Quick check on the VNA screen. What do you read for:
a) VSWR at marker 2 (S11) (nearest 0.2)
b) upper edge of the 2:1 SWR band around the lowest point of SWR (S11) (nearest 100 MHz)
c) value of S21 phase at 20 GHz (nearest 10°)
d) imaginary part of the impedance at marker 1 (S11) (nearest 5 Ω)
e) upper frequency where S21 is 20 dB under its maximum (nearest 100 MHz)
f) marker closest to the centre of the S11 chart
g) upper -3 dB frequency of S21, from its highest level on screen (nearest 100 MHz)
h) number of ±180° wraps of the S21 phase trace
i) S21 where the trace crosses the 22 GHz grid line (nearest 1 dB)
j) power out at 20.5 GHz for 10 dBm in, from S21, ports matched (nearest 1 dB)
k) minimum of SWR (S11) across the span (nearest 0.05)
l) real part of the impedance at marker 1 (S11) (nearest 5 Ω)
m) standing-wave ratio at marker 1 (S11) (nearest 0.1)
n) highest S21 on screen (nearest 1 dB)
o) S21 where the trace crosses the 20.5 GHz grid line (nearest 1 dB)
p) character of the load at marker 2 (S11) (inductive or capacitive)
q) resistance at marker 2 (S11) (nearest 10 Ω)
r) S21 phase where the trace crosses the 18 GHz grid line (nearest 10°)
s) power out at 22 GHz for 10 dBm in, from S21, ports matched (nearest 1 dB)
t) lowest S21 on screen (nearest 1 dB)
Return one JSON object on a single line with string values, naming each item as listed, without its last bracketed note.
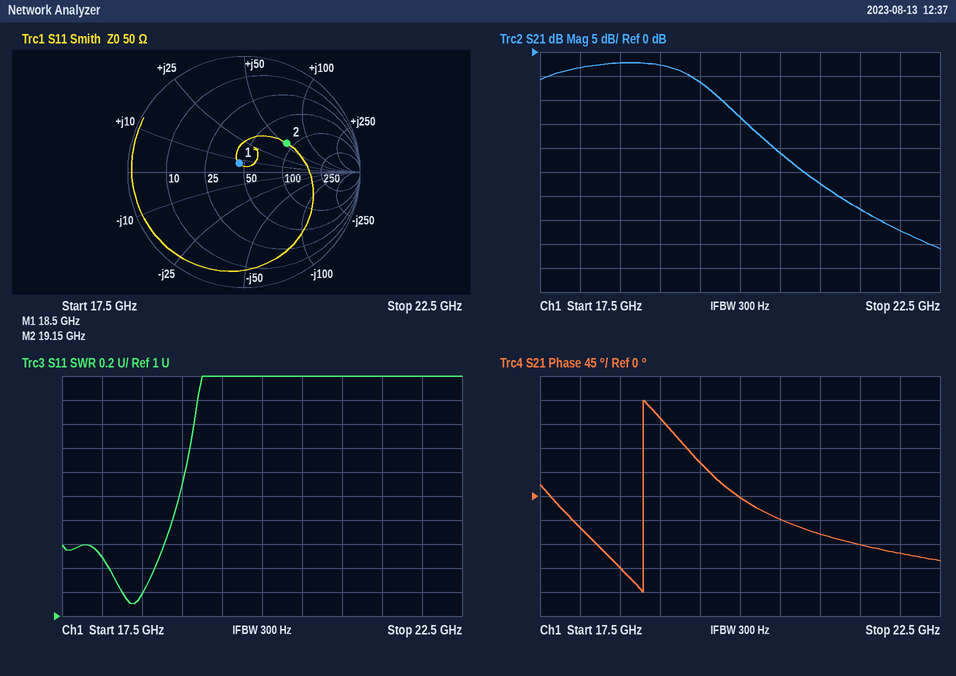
{"VSWR at marker 2 (S11)": "2.6", "upper edge of the 2:1 SWR band around the lowest point of SWR (S11)": "19.0 GHz", "value of S21 phase at 20 GHz": "0°", "imaginary part of the impedance at marker 1 (S11)": "+5 Ω", "upper frequency where S21 is 20 dB under its maximum": "20.6 GHz", "marker closest to the centre of the S11 chart": "marker 1", "upper -3 dB frequency of S21, from its highest level on screen": "19.4 GHz", "number of ±180° wraps of the S21 phase trace": "1", "S21 where the trace crosses the 22 GHz grid line": "-37 dB", "power out at 20.5 GHz for 10 dBm in, from S21, ports matched": "-11 dBm", "minimum of SWR (S11) across the span": "1.10", "real part of the impedance at marker 1 (S11)": "45 Ω", "standing-wave ratio at marker 1 (S11)": "1.2", "highest S21 on screen": "-2 dB", "S21 where the trace crosses the 20.5 GHz grid line": "-21 dB", "character of the load at marker 2 (S11)": "inductive", "resistance at marker 2 (S11)": "90 Ω", "S21 phase where the trace crosses the 18 GHz grid line": "-60°", "power out at 22 GHz for 10 dBm in, from S21, ports matched": "-27 dBm", "lowest S21 on screen": "-41 dB"}
